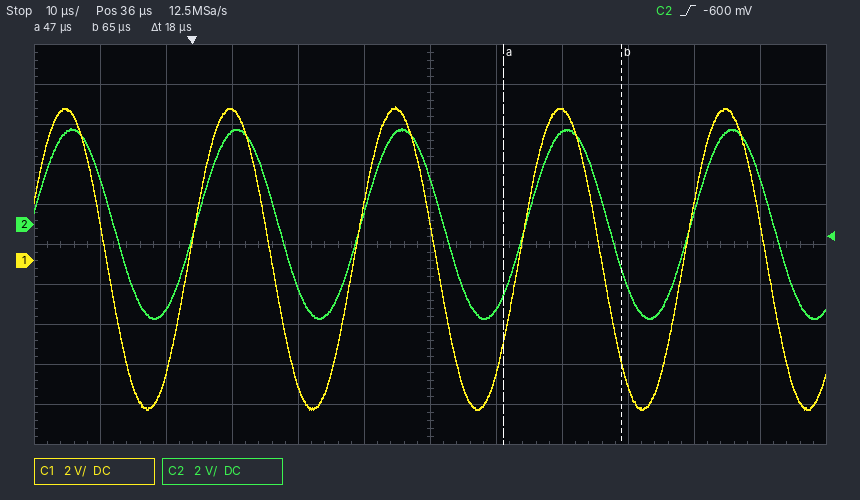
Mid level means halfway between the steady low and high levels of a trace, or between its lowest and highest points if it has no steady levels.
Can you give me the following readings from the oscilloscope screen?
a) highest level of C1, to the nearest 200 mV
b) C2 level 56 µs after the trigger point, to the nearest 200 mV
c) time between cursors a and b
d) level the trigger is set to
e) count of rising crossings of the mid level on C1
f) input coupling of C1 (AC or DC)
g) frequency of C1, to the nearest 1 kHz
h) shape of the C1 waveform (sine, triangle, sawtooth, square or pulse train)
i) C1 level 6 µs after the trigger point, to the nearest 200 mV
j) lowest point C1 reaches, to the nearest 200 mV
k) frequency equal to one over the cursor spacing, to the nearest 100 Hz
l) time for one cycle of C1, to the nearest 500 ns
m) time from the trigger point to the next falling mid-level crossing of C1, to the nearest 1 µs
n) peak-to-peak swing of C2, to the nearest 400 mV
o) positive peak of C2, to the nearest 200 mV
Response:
7.6 V
4.6 V
18 µs
-600 mV
4
DC
40 kHz
sine
7.6 V
-7.4 V
55.6 kHz
25.0 µs
12 µs
9.6 V
4.8 V
